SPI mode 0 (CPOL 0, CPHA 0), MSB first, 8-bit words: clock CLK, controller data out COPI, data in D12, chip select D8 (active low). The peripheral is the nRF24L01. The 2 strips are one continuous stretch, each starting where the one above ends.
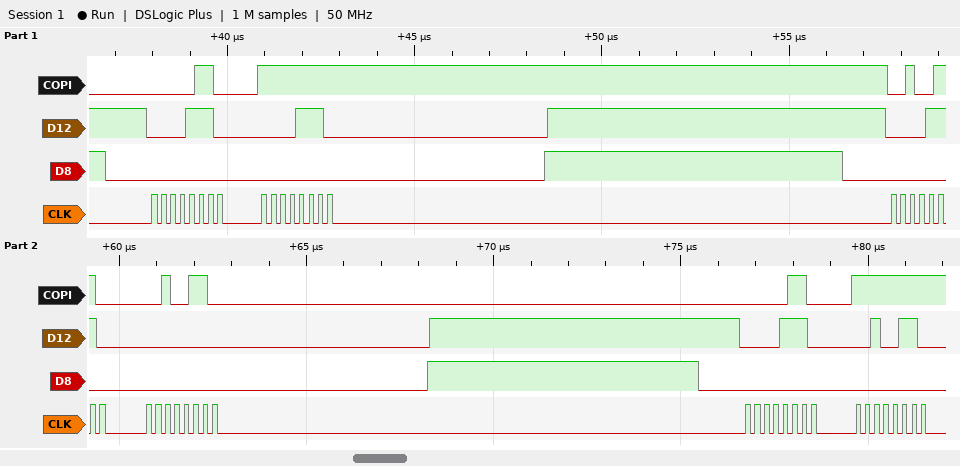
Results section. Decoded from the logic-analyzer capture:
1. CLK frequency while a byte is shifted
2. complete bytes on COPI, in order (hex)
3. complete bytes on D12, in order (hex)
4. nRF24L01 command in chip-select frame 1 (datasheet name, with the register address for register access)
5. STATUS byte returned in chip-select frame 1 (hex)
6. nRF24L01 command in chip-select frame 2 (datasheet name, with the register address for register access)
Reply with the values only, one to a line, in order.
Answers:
4 MHz
06 FF 26 26 06 FF
0E 0E 0E 00 0E 26
R_REGISTER 0x06
0x0E
W_REGISTER 0x06
